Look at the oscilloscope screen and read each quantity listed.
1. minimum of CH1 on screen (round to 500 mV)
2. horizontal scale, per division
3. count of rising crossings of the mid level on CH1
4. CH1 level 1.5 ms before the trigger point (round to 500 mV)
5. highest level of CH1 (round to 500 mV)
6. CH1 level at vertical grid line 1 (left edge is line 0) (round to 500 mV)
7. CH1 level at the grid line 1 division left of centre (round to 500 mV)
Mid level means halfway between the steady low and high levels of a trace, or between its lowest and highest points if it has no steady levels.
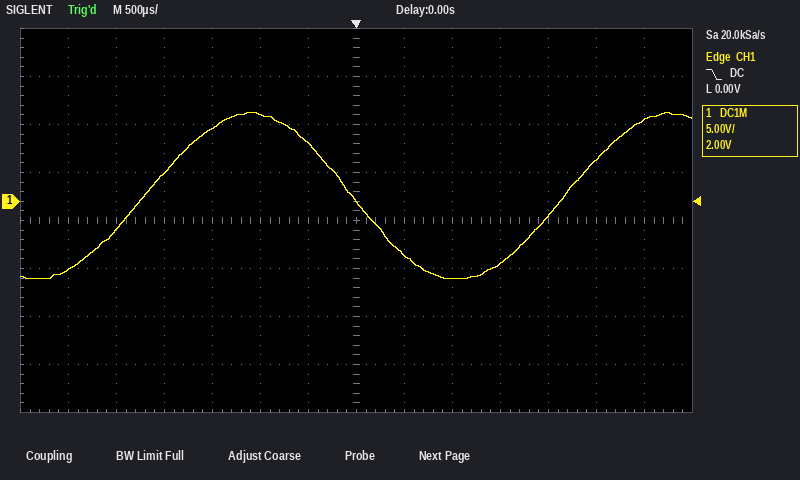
-8.0 V
500 µs
2
7.5 V
9.0 V
-7.0 V
6.0 V
